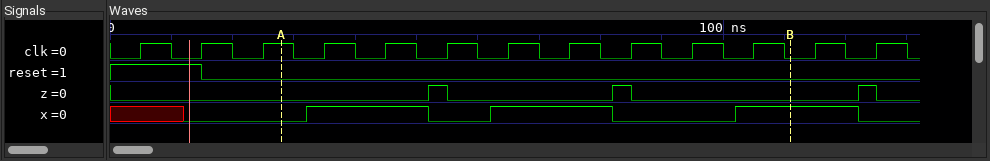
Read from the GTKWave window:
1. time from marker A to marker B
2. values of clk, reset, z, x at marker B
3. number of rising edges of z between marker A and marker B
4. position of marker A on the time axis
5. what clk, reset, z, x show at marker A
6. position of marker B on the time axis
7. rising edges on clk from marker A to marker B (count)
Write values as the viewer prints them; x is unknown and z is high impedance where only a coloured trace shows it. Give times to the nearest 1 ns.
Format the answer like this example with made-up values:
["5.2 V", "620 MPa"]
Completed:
["83 ns", "clk=0, reset=0, z=0, x=1", "2", "28 ns", "clk=1, reset=0, z=0, x=0", "111 ns", "8"]
